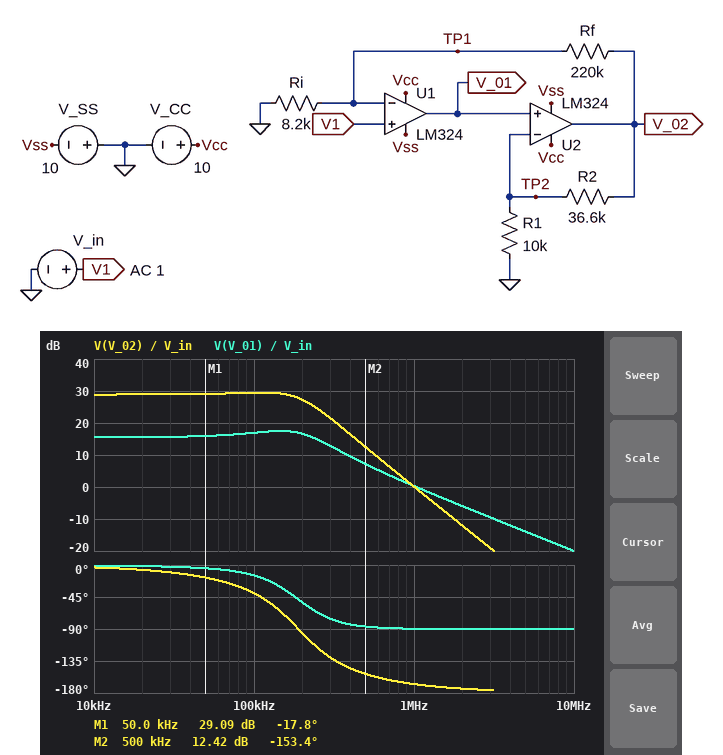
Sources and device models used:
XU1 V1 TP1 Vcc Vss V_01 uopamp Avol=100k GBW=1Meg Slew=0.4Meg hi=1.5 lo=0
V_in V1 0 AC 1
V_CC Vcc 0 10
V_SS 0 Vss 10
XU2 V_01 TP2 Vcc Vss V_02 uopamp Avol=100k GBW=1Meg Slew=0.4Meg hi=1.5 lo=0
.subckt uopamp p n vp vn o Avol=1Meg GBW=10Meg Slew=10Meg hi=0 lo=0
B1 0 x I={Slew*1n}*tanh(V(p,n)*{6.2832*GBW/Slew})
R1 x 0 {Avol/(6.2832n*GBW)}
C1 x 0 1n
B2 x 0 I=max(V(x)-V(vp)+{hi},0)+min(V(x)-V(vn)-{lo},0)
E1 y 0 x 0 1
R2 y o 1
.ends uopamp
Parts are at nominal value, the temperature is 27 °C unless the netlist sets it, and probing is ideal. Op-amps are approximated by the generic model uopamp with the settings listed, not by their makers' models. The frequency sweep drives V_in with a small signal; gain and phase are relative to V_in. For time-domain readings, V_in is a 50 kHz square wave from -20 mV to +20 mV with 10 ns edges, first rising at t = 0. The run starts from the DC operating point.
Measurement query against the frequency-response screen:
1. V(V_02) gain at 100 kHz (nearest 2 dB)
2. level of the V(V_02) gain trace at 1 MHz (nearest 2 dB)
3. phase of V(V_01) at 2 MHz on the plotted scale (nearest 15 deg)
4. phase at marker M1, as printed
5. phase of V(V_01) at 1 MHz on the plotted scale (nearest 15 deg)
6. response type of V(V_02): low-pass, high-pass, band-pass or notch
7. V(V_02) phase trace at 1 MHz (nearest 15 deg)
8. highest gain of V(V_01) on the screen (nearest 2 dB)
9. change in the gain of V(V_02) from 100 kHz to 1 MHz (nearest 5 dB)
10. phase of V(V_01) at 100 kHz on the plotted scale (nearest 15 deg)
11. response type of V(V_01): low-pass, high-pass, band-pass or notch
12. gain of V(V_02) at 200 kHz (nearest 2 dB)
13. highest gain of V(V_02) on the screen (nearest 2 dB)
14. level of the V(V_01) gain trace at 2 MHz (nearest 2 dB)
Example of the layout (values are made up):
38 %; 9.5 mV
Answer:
30 dB; 0 dB; -90 deg; -17.8 deg; -90 deg; low-pass; -165 deg; 18 dB; -30 dB; -15 deg; low-pass; 28 dB; 30 dB; -6 dB
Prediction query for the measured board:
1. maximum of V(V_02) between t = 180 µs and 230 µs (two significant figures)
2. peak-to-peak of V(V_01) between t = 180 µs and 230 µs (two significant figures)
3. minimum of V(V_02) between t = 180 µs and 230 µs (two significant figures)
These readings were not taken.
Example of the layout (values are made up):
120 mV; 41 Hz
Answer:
920 mV; 530 mV; -920 mV
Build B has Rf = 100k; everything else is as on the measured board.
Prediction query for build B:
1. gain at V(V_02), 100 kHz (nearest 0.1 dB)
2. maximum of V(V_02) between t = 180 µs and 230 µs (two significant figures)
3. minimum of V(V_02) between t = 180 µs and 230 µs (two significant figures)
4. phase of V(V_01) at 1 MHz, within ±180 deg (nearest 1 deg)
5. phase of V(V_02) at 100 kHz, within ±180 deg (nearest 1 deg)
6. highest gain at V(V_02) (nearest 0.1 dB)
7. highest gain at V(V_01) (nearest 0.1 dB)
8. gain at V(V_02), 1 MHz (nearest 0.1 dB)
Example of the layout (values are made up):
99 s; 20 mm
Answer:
23.2 dB; 470 mV; -470 mV; -89 deg; -18 deg; 25.3 dB; 15.5 dB; 0.5 dB
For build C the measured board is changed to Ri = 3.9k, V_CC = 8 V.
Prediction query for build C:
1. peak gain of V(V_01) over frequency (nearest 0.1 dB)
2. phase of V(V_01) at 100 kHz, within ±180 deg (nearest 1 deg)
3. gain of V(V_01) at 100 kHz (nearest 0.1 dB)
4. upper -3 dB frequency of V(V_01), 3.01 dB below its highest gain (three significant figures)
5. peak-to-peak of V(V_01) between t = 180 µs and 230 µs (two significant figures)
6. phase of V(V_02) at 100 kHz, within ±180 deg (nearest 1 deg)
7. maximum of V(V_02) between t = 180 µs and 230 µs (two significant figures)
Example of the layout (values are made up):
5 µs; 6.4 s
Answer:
21.8 dB; -46 deg; 20.4 dB; 136 kHz; 1.6 V; -71 deg; 1.9 V
